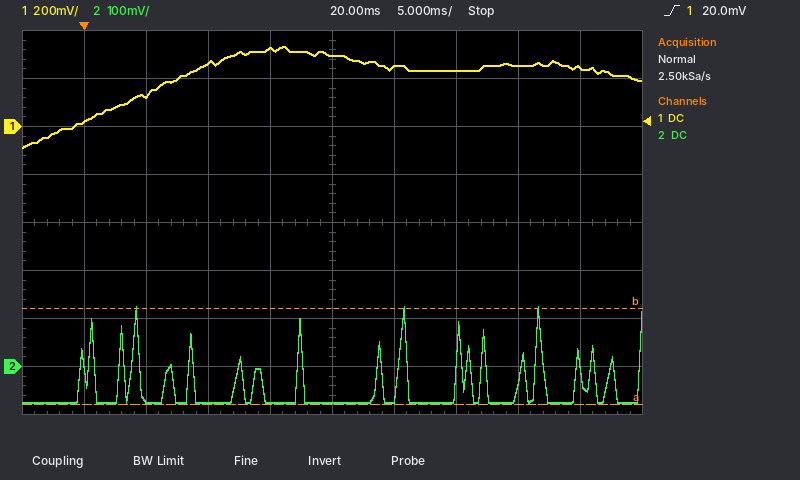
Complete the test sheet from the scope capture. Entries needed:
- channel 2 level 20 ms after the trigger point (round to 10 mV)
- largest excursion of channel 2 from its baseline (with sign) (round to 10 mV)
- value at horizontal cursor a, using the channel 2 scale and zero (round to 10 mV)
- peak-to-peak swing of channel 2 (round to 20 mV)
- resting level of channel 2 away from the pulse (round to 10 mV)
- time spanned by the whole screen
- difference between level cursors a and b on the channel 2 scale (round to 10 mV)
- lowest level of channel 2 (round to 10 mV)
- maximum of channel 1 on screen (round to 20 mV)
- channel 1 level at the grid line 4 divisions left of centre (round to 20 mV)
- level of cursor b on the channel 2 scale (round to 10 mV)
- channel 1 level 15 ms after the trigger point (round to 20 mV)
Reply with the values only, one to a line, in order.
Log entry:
-80 mV
+200 mV
-80 mV
200 mV
-80 mV
50 ms
200 mV
-80 mV
340 mV
20 mV
120 mV
320 mV
